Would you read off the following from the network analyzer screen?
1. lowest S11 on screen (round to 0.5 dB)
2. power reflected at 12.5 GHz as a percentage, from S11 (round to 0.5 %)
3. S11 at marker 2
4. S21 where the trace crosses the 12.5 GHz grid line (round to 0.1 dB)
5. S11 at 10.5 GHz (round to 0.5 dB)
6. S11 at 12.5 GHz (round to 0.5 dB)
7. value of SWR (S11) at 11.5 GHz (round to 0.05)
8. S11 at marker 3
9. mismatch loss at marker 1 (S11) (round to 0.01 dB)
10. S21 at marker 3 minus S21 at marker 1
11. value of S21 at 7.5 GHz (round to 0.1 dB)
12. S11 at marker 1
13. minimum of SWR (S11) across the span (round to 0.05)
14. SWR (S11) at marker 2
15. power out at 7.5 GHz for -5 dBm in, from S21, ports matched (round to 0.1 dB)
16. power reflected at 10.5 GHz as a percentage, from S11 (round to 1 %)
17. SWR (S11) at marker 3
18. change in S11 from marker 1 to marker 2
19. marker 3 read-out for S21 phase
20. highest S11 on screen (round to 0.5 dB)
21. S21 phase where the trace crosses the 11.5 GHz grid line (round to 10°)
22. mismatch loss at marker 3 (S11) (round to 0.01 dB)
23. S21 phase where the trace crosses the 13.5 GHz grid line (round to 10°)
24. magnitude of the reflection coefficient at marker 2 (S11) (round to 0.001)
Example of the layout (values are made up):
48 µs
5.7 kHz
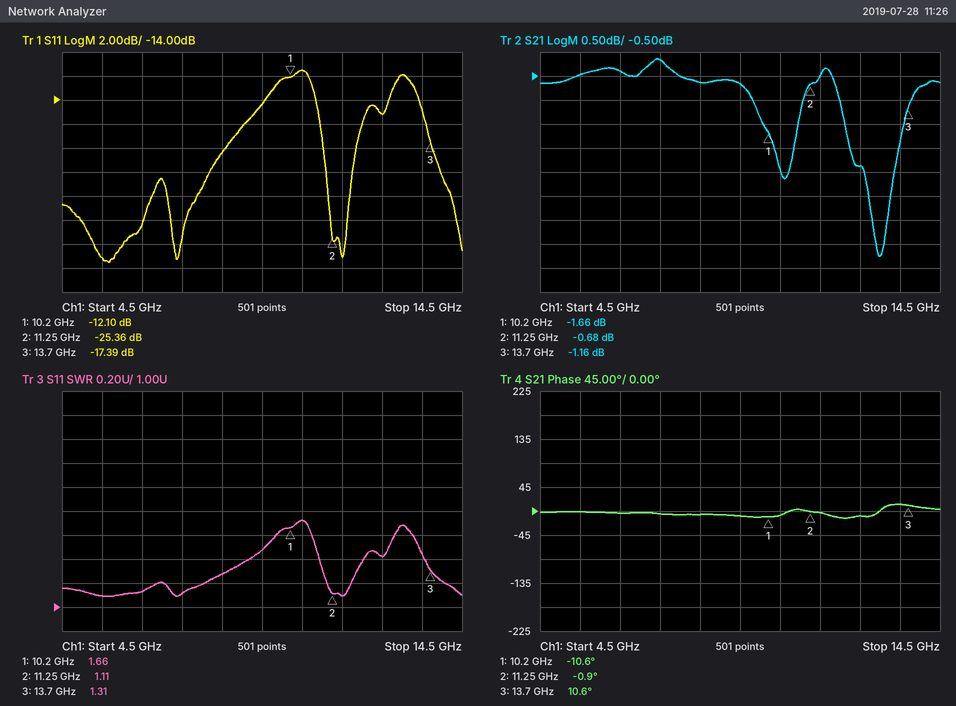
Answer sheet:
-27.5 dB
3.0 %
-25.36 dB
-2.4 dB
-11.5 dB
-15.0 dB
1.10
-17.39 dB
0.28 dB
0.50 dB
-0.2 dB
-12.10 dB
1.10
1.11
-5.2 dBm
7 %
1.31
-13.26 dB
10.6°
-11.5 dB
0°
0.08 dB
10°
0.054
